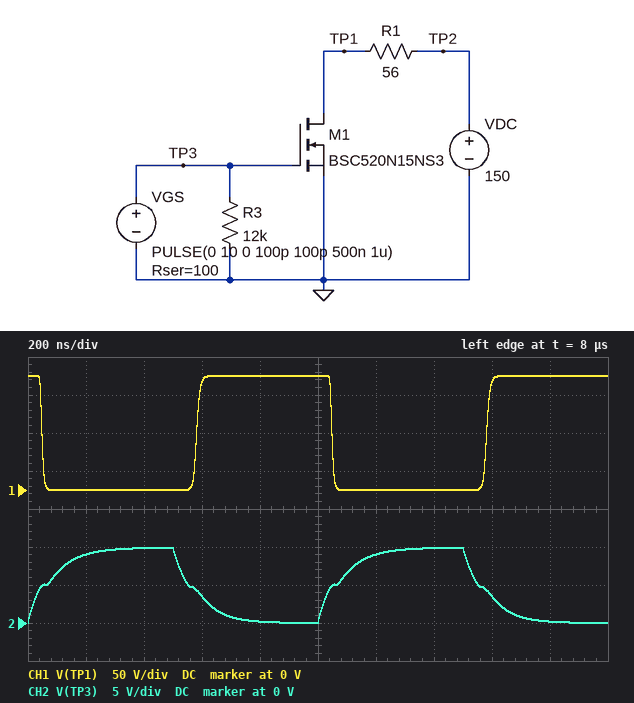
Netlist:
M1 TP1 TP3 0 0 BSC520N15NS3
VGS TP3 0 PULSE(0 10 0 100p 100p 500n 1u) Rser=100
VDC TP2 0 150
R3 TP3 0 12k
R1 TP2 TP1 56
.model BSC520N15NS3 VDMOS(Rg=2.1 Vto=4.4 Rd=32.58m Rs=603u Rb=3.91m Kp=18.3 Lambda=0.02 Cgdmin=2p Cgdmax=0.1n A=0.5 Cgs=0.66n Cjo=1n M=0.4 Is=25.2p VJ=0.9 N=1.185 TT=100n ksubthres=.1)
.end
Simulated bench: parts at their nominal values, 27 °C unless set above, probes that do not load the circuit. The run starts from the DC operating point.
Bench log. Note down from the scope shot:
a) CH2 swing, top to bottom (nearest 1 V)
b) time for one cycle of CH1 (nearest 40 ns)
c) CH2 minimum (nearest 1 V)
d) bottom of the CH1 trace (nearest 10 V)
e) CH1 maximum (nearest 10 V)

10 V
1.00 µs
0 V
0 V
150 V
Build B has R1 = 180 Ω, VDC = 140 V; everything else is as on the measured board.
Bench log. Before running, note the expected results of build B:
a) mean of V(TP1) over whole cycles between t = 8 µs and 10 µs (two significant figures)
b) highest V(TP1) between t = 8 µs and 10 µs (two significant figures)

62 V
140 V
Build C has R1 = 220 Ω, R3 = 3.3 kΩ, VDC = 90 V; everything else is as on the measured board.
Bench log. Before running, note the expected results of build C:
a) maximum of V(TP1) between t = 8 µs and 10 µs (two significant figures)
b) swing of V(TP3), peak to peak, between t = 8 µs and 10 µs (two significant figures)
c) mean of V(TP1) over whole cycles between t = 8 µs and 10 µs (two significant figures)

90 V
9.7 V
39 V
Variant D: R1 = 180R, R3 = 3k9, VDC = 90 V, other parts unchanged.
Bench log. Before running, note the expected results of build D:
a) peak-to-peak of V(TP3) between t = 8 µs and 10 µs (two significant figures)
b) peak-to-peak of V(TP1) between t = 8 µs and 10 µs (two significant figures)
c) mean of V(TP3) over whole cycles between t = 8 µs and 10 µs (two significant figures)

9.7 V
90 V
4.9 V
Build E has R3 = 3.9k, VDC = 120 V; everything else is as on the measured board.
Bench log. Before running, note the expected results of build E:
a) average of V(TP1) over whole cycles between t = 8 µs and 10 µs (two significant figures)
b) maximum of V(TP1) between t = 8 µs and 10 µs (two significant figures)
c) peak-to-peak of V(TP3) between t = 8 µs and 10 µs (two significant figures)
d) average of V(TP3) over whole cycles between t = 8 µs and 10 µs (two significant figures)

56 V
120 V
9.7 V
4.9 V
